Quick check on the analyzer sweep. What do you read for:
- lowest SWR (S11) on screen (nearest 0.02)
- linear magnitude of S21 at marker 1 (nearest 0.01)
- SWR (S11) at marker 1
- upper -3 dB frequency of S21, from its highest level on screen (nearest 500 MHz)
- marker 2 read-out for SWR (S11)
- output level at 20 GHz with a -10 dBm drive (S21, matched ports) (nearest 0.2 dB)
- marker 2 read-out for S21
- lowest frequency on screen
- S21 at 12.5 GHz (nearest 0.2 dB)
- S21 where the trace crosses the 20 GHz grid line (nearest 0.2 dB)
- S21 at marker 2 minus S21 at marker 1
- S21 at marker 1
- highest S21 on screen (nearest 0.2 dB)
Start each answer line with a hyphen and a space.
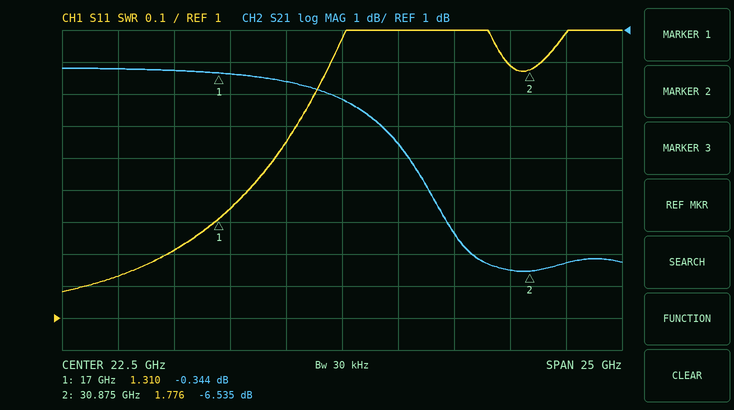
- 1.08
- 0.96
- 1.310
- 25.5 GHz
- 1.776
- -10.6 dBm
- -6.535 dB
- 10 GHz
- -0.2 dB
- -0.6 dB
- -6.191 dB
- -0.344 dB
- -0.2 dB
